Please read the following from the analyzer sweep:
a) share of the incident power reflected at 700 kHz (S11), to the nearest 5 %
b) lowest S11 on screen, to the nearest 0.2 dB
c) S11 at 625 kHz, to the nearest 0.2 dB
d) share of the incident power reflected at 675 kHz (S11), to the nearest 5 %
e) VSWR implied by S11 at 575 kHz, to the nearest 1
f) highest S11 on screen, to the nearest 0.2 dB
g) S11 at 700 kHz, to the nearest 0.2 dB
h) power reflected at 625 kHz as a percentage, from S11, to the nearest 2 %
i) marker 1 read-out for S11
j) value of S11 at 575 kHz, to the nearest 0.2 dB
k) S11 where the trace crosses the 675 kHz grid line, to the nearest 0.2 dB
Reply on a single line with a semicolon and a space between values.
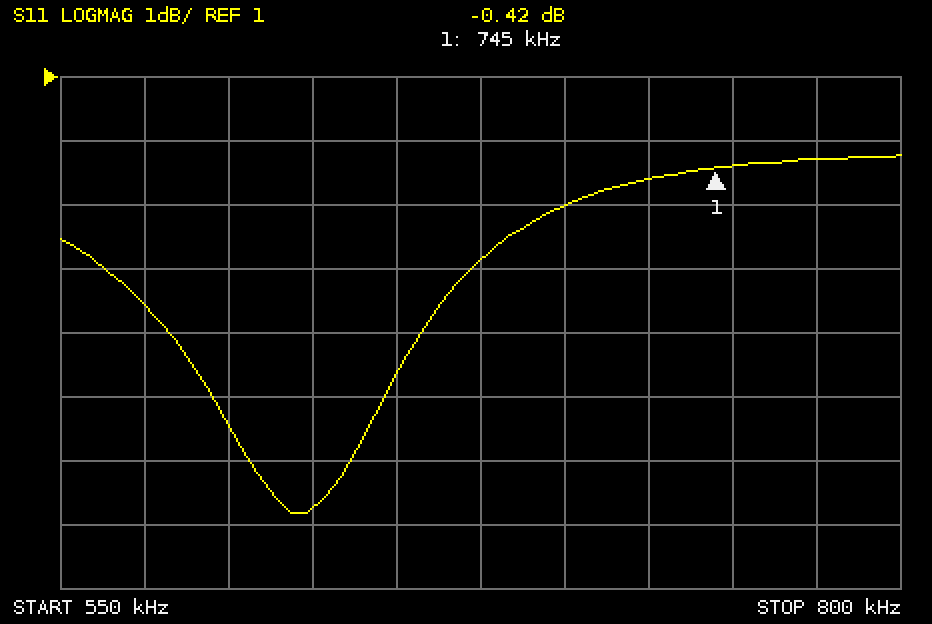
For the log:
80 %; -5.8 dB; -5.8 dB; 65 %; 7; -0.2 dB; -1.0 dB; 26 %; -0.42 dB; -2.6 dB; -1.8 dB
